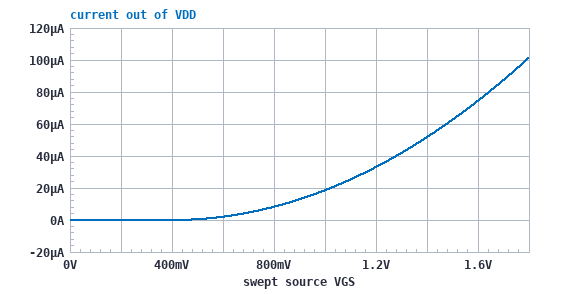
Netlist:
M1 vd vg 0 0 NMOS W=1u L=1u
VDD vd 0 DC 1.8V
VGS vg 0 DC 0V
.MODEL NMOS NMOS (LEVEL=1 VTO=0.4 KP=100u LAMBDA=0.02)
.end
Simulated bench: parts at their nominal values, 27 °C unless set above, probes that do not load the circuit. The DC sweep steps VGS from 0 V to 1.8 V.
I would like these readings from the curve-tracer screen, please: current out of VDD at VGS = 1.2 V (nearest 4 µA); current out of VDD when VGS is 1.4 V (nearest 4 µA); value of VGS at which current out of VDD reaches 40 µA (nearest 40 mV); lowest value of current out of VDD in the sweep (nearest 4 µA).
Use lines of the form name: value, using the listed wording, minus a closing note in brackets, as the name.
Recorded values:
current out of VDD at VGS = 1.2 V: 32 µA
current out of VDD when VGS is 1.4 V: 52 µA
value of VGS at which current out of VDD reaches 40 µA: 1.28 V
lowest value of current out of VDD in the sweep: 0 A
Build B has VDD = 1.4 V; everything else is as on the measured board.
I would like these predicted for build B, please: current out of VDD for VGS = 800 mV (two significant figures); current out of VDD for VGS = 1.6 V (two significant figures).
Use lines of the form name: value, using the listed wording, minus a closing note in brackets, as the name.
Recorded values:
current out of VDD for VGS = 800 mV: 8.2 µA
current out of VDD for VGS = 1.6 V: 74 µA
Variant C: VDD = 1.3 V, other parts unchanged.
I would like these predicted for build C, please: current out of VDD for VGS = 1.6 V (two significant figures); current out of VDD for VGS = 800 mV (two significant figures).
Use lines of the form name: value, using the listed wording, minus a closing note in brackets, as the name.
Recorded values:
current out of VDD for VGS = 1.6 V: 74 µA
current out of VDD for VGS = 800 mV: 8.2 µA
